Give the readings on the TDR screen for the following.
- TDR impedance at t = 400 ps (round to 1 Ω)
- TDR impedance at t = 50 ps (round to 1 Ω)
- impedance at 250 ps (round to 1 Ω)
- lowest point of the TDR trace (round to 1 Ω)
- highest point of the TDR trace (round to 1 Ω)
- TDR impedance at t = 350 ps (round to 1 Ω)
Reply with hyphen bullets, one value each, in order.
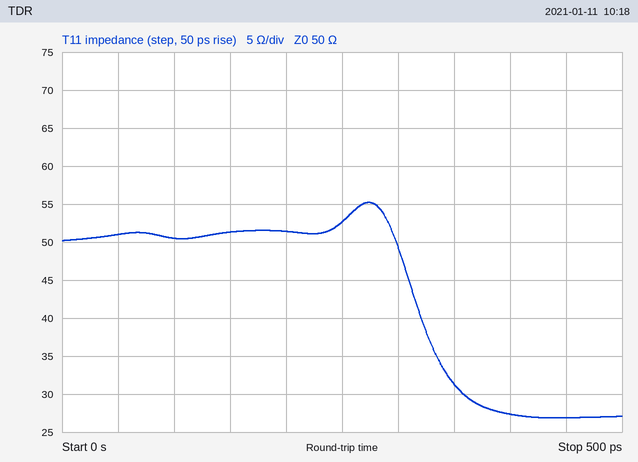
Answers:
- 27 Ω
- 51 Ω
- 53 Ω
- 27 Ω
- 55 Ω
- 31 Ω
